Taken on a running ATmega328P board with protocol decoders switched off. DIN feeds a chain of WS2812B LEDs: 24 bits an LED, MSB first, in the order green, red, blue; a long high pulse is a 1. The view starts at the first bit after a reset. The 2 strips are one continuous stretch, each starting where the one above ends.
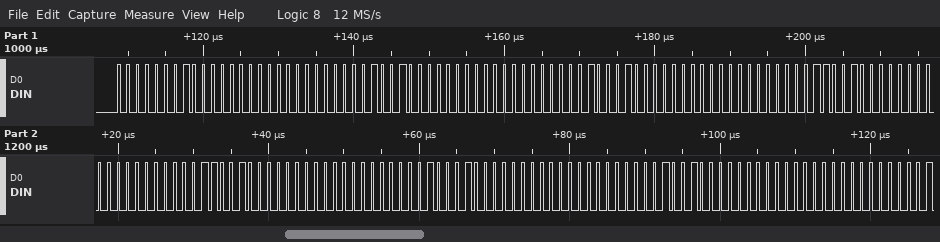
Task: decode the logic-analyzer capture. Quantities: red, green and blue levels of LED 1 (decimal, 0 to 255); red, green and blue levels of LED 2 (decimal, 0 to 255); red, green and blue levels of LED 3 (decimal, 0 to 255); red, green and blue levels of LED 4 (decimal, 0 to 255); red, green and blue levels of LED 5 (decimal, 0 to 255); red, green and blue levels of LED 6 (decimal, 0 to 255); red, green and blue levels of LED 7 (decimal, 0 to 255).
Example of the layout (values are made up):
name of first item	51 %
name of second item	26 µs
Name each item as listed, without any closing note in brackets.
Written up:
red, green and blue levels of LED 1	0, 1, 0
red, green and blue levels of LED 2	0, 18, 0
red, green and blue levels of LED 3	0, 34, 0
red, green and blue levels of LED 4	0, 50, 0
red, green and blue levels of LED 5	0, 50, 0
red, green and blue levels of LED 6	0, 34, 0
red, green and blue levels of LED 7	0, 18, 0
